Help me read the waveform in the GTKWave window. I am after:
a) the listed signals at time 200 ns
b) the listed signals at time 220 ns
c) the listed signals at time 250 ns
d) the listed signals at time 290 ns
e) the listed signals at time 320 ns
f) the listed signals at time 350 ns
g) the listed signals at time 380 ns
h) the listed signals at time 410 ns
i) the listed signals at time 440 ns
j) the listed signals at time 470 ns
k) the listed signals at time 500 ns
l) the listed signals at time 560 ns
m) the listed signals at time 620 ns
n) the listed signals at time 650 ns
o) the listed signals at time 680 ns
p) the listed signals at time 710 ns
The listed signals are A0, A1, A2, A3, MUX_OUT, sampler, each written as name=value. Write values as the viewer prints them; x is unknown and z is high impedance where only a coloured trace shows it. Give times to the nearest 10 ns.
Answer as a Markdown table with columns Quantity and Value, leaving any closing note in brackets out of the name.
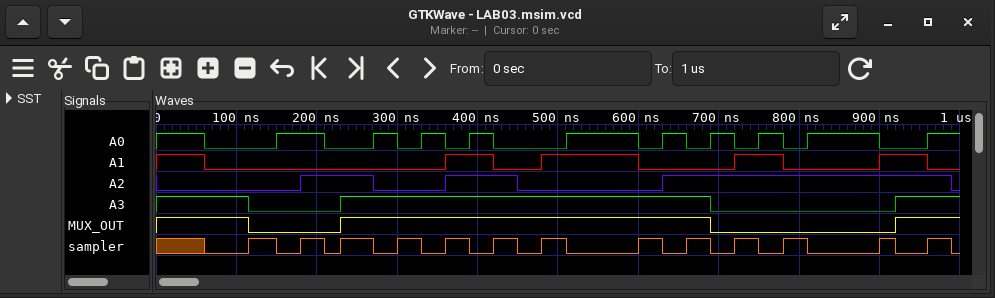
| Quantity | Value |
|---|---|
| the listed signals at time 200 ns | A0=1, A1=0, A2=1, A3=0, MUX_OUT=0, sampler=1 |
| the listed signals at time 220 ns | A0=0, A1=0, A2=1, A3=0, MUX_OUT=0, sampler=0 |
| the listed signals at time 250 ns | A0=0, A1=0, A2=1, A3=1, MUX_OUT=1, sampler=1 |
| the listed signals at time 290 ns | A0=1, A1=0, A2=0, A3=1, MUX_OUT=1, sampler=0 |
| the listed signals at time 320 ns | A0=0, A1=0, A2=0, A3=1, MUX_OUT=1, sampler=1 |
| the listed signals at time 350 ns | A0=1, A1=0, A2=0, A3=1, MUX_OUT=1, sampler=0 |
| the listed signals at time 380 ns | A0=0, A1=1, A2=1, A3=1, MUX_OUT=1, sampler=1 |
| the listed signals at time 410 ns | A0=1, A1=1, A2=1, A3=1, MUX_OUT=1, sampler=0 |
| the listed signals at time 440 ns | A0=0, A1=0, A2=1, A3=1, MUX_OUT=1, sampler=1 |
| the listed signals at time 470 ns | A0=0, A1=0, A2=0, A3=1, MUX_OUT=1, sampler=0 |
| the listed signals at time 500 ns | A0=0, A1=1, A2=0, A3=1, MUX_OUT=1, sampler=1 |
| the listed signals at time 560 ns | A0=1, A1=1, A2=0, A3=1, MUX_OUT=1, sampler=0 |
| the listed signals at time 620 ns | A0=0, A1=0, A2=0, A3=1, MUX_OUT=1, sampler=1 |
| the listed signals at time 650 ns | A0=1, A1=0, A2=1, A3=1, MUX_OUT=1, sampler=0 |
| the listed signals at time 680 ns | A0=0, A1=0, A2=1, A3=1, MUX_OUT=1, sampler=1 |
| the listed signals at time 710 ns | A0=1, A1=0, A2=1, A3=0, MUX_OUT=0, sampler=0 |
